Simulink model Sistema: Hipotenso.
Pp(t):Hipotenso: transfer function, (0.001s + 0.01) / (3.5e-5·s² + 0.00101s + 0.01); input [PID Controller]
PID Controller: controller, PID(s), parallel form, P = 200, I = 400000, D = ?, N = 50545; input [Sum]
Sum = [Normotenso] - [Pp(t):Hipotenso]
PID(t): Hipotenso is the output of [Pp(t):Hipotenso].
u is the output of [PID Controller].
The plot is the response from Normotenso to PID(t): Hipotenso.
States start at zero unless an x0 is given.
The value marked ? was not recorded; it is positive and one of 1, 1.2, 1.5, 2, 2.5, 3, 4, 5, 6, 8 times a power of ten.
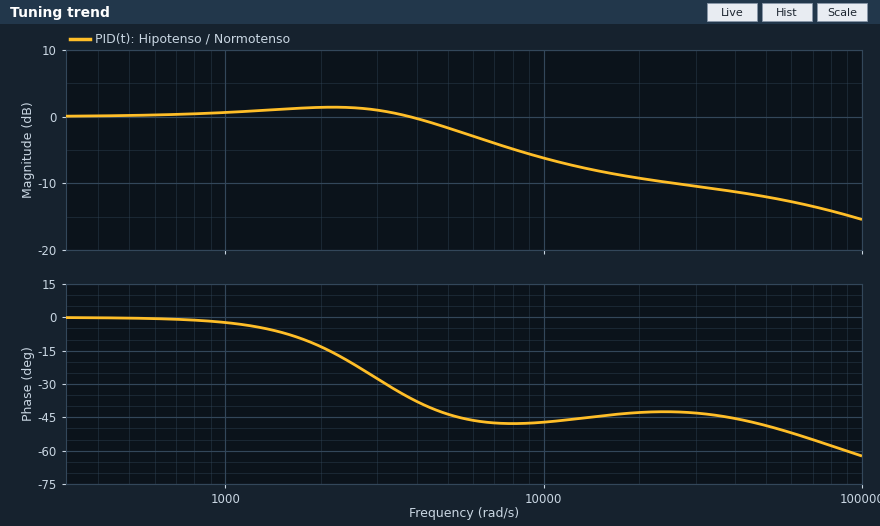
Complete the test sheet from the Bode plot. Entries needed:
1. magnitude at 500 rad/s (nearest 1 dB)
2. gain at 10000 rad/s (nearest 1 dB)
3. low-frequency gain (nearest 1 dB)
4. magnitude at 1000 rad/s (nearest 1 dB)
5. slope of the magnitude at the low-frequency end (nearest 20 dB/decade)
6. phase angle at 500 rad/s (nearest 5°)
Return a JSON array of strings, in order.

["0 dB", "-6 dB", "0 dB", "1 dB", "0 dB/decade", "0°"]
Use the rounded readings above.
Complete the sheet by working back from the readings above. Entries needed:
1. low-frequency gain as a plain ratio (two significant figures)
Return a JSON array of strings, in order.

["1.0"]
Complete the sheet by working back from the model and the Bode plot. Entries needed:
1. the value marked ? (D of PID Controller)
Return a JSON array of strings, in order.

["0.01"]
